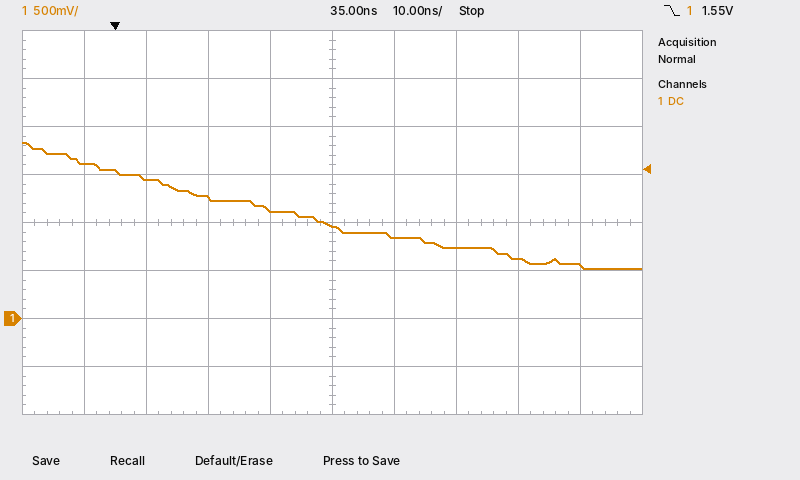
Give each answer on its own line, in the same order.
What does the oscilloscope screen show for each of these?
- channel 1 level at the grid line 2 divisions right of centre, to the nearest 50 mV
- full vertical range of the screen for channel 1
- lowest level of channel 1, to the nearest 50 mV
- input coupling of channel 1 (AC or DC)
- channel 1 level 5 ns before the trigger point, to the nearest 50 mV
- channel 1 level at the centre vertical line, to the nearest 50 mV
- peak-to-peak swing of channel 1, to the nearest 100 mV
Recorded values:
750 mV
4 V
500 mV
DC
1.60 V
950 mV
1.30 V
